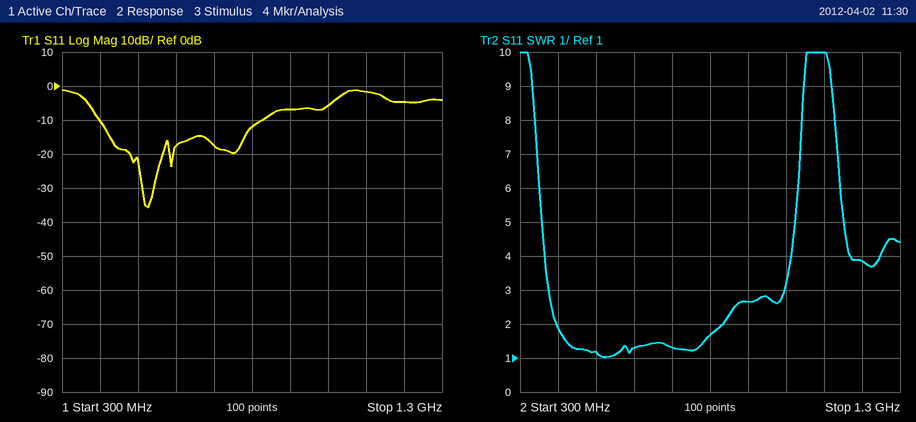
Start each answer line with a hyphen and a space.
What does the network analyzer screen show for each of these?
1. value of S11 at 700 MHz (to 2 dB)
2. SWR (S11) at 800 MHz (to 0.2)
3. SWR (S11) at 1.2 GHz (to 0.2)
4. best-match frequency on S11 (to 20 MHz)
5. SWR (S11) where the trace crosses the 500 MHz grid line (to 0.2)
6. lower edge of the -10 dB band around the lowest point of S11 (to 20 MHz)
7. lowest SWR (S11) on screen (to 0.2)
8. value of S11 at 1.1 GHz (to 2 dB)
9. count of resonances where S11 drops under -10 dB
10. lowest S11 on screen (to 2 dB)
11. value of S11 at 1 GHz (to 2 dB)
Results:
- -18 dB
- 1.6
- 3.8
- 520 MHz
- 1.2
- 400 MHz
- 1.0
- -2 dB
- 3
- -36 dB
- -6 dB
